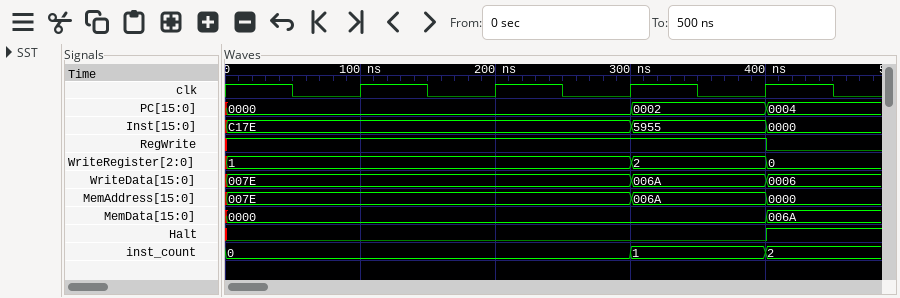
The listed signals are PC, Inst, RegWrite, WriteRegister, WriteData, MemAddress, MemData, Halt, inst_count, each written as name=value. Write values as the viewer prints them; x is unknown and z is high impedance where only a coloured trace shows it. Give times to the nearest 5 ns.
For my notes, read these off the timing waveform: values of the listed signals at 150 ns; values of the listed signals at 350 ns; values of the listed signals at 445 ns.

PC=0000, Inst=C17E, RegWrite=1, WriteRegister=1, WriteData=007E, MemAddress=007E, MemData=0000, Halt=0, inst_count=0
PC=0002, Inst=5955, RegWrite=1, WriteRegister=2, WriteData=006A, MemAddress=006A, MemData=0000, Halt=0, inst_count=1
PC=0004, Inst=0000, RegWrite=0, WriteRegister=0, WriteData=0006, MemAddress=0000, MemData=006A, Halt=1, inst_count=2
